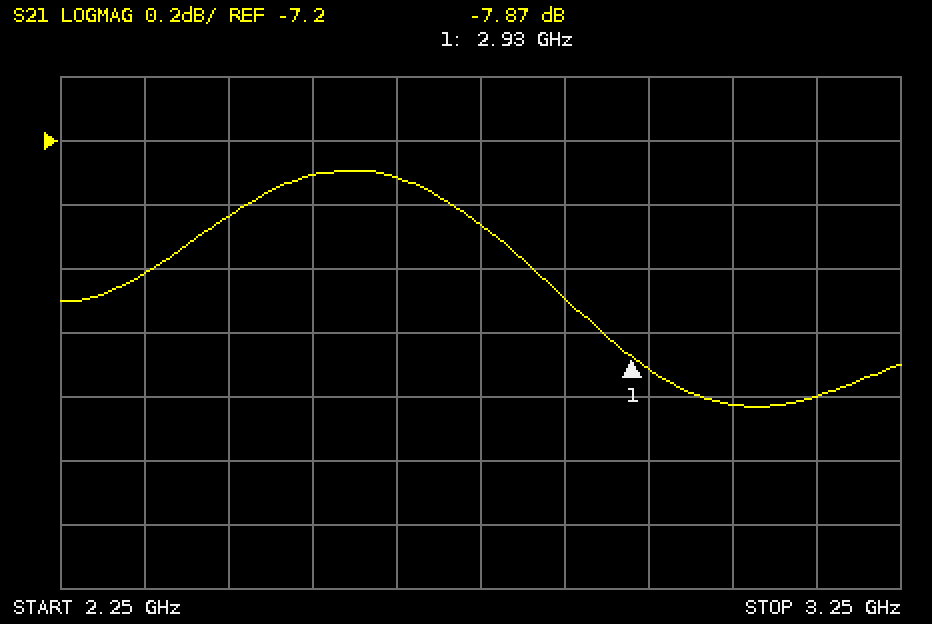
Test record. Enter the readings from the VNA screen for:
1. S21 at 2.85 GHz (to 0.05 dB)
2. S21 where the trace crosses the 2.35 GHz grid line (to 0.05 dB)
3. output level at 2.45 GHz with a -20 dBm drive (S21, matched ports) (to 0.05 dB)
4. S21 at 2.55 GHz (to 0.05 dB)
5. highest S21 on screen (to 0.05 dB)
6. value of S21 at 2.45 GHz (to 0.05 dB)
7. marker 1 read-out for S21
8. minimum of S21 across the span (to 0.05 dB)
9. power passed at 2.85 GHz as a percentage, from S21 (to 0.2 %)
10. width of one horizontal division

-7.70 dB
-7.60 dB
-27.45 dBm
-7.30 dB
-7.30 dB
-7.45 dB
-7.87 dB
-8.05 dB
17.0 %
100 MHz
